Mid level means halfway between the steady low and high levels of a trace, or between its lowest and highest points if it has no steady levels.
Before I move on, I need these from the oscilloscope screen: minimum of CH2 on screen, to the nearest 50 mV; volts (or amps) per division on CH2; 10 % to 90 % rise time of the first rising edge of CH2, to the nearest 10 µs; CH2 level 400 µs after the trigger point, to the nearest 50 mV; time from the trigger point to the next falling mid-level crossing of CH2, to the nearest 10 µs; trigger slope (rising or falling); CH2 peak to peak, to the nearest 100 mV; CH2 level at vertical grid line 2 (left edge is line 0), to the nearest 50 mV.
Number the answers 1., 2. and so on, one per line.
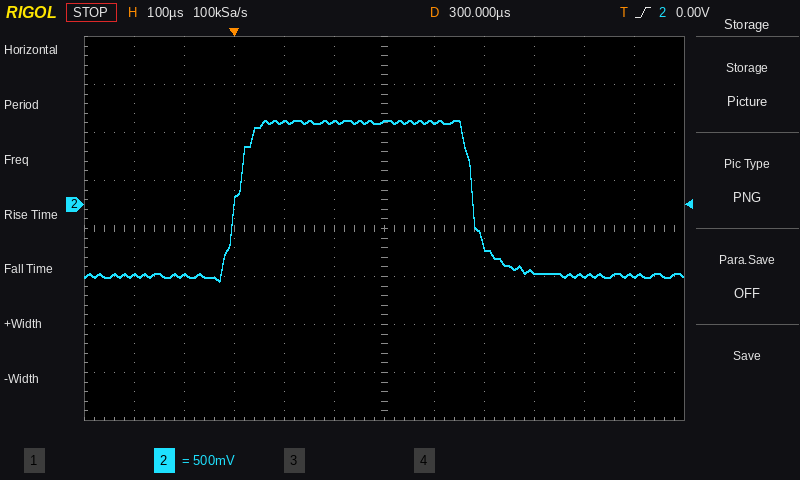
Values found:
1. -800 mV
2. 500 mV
3. 60 µs
4. 850 mV
5. 480 µs
6. rising
7. 1.70 V
8. -750 mV
